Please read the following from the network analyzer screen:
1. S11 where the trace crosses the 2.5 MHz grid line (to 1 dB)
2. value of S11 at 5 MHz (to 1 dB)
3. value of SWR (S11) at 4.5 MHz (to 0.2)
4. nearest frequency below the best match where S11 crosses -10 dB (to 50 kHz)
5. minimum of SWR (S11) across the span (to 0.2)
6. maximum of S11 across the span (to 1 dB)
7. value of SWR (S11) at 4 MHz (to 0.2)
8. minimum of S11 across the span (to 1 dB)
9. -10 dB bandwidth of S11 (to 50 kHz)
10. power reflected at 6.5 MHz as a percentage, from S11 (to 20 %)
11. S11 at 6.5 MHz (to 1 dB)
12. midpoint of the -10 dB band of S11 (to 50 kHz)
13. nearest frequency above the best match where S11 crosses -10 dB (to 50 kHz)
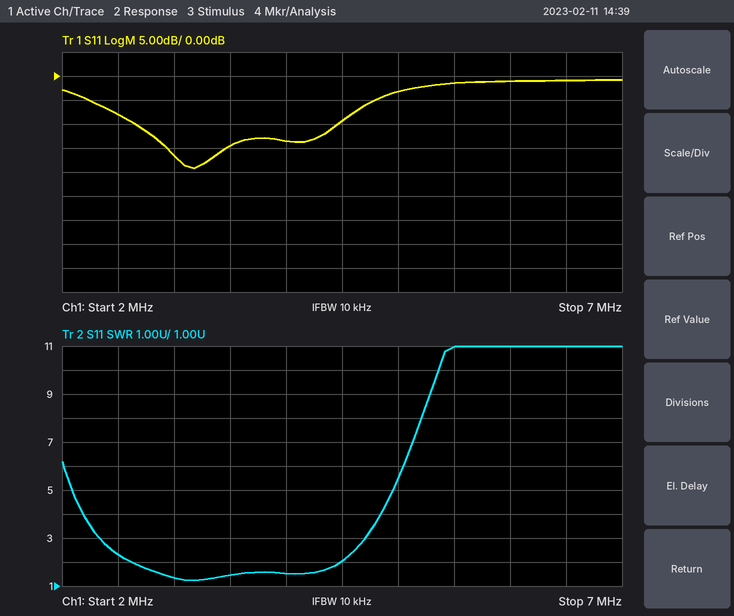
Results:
-8 dB
-3 dB
2.0
2.65 MHz
1.2
-1 dB
1.6
-19 dB
1.80 MHz
80 %
-1 dB
3.55 MHz
4.45 MHz
